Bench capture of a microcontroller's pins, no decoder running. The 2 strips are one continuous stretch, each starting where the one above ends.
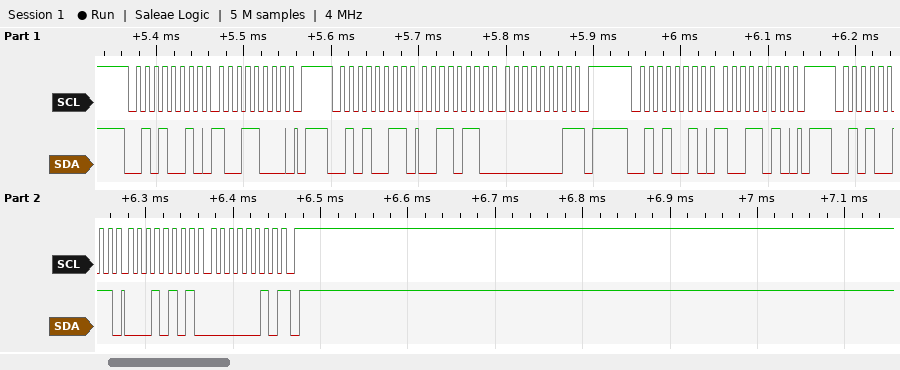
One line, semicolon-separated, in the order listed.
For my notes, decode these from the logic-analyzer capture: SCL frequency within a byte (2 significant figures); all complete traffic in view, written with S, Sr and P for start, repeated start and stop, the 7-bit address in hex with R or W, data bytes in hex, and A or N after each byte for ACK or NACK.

100 kHz; S 29W A 98 A P S 29R A 36 A 01 N P S 29W A 9A A P S 29R A 15 A 02 N P
